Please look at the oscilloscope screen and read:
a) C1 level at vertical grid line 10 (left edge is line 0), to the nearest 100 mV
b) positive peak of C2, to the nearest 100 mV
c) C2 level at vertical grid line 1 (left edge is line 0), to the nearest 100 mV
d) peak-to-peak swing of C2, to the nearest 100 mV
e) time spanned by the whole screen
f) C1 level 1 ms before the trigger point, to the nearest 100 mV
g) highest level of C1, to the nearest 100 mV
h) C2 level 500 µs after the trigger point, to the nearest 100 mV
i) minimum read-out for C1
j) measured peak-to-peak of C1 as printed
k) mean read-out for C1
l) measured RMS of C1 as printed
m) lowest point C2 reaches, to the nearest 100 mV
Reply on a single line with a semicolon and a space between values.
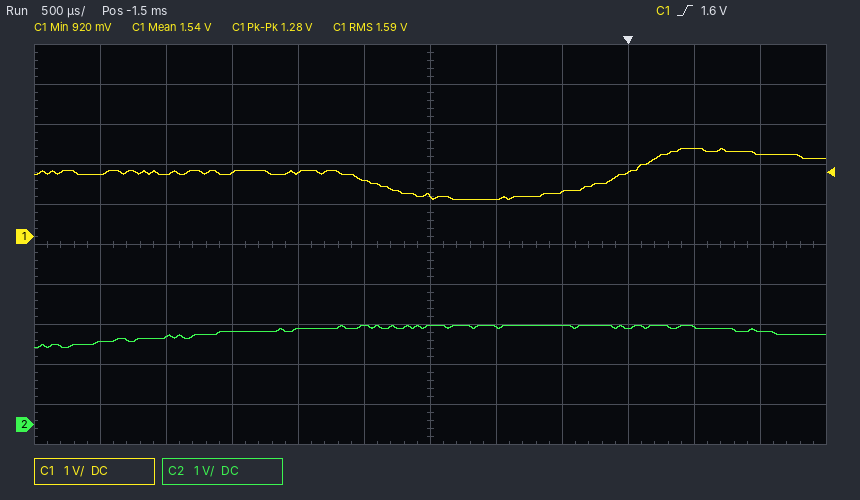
2.2 V; 2.5 V; 2.1 V; 600 mV; 6 ms; 900 mV; 2.2 V; 2.4 V; 920 mV; 1.28 V; 1.54 V; 1.59 V; 1.9 V
